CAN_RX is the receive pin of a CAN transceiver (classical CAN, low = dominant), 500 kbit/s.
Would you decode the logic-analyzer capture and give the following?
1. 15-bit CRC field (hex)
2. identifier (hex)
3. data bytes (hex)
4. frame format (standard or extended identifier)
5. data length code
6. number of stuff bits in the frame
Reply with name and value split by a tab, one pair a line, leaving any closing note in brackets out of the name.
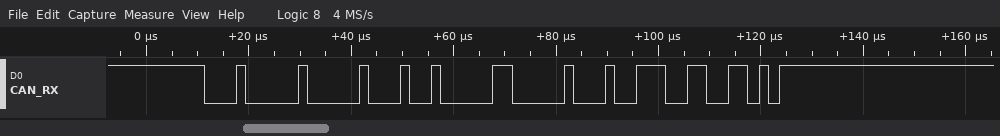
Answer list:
15-bit CRC field	0x4E66
identifier	0x100
data bytes	41 00
frame format	standard
data length code	2
number of stuff bits in the frame	4
